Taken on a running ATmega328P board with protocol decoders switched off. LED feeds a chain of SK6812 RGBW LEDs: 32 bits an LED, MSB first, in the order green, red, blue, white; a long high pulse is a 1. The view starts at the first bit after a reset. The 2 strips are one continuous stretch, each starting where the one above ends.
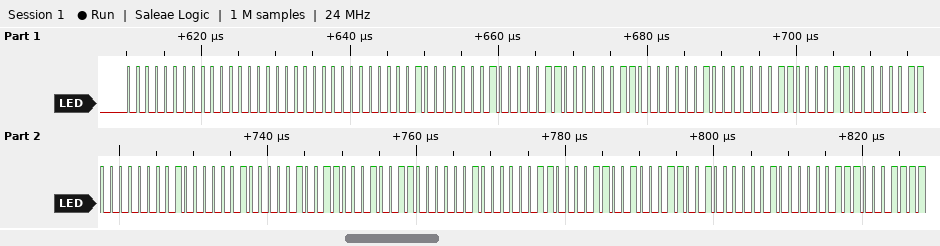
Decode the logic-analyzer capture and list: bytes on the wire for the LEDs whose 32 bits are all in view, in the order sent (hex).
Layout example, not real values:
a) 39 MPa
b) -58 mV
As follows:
a) 00 00 00 01 01 06 06 02 03 0C 0C 02 04 13 13 02 06 19 19 02
